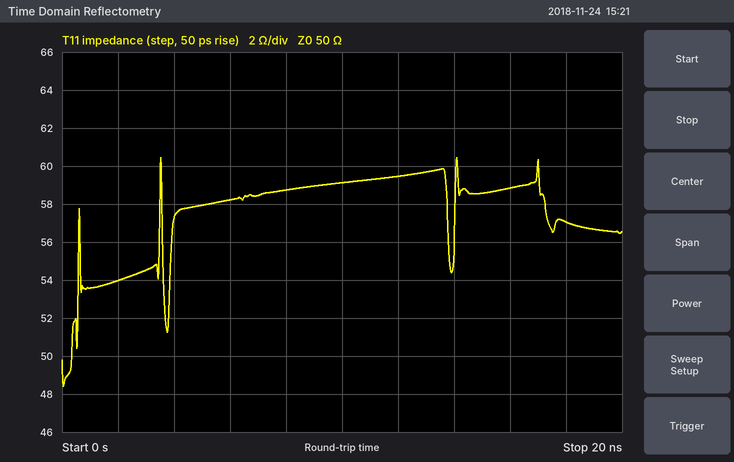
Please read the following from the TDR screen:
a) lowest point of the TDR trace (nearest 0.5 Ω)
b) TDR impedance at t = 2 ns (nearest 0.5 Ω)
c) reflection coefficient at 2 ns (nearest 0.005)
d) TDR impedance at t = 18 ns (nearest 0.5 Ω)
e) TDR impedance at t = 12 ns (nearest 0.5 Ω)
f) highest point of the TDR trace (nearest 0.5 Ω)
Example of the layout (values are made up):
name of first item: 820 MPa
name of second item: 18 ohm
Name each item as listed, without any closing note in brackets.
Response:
lowest point of the TDR trace: 48.5 Ω
TDR impedance at t = 2 ns: 54.0 Ω
reflection coefficient at 2 ns: +0.040
TDR impedance at t = 18 ns: 57.0 Ω
TDR impedance at t = 12 ns: 59.5 Ω
highest point of the TDR trace: 60.5 Ω
